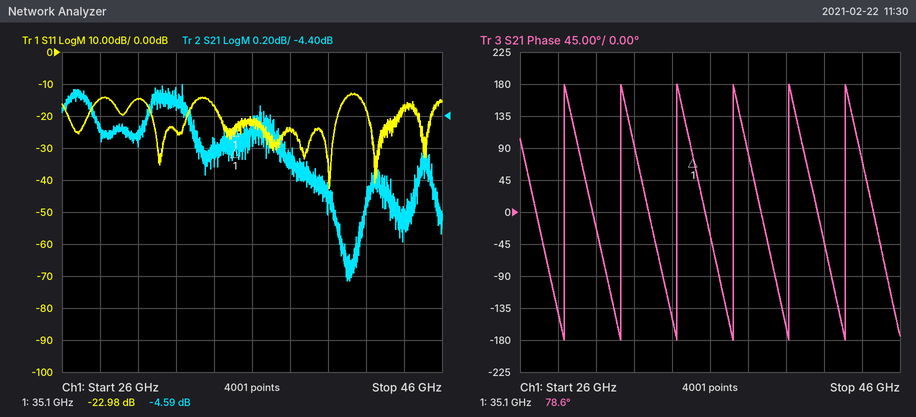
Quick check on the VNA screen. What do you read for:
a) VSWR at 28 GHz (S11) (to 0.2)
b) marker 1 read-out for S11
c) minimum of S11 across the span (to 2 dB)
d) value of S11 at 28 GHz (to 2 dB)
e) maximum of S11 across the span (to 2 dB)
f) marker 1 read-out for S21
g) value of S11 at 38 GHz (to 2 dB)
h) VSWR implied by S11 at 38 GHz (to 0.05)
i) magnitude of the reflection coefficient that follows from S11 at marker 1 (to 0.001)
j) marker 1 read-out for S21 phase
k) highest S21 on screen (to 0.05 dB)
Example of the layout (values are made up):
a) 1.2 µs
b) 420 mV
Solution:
a) 1.4
b) -22.98 dB
c) -42 dB
d) -14 dB
e) -12 dB
f) -4.59 dB
g) -24 dB
h) 1.15
i) 0.071
j) 78.6°
k) -4.20 dB
